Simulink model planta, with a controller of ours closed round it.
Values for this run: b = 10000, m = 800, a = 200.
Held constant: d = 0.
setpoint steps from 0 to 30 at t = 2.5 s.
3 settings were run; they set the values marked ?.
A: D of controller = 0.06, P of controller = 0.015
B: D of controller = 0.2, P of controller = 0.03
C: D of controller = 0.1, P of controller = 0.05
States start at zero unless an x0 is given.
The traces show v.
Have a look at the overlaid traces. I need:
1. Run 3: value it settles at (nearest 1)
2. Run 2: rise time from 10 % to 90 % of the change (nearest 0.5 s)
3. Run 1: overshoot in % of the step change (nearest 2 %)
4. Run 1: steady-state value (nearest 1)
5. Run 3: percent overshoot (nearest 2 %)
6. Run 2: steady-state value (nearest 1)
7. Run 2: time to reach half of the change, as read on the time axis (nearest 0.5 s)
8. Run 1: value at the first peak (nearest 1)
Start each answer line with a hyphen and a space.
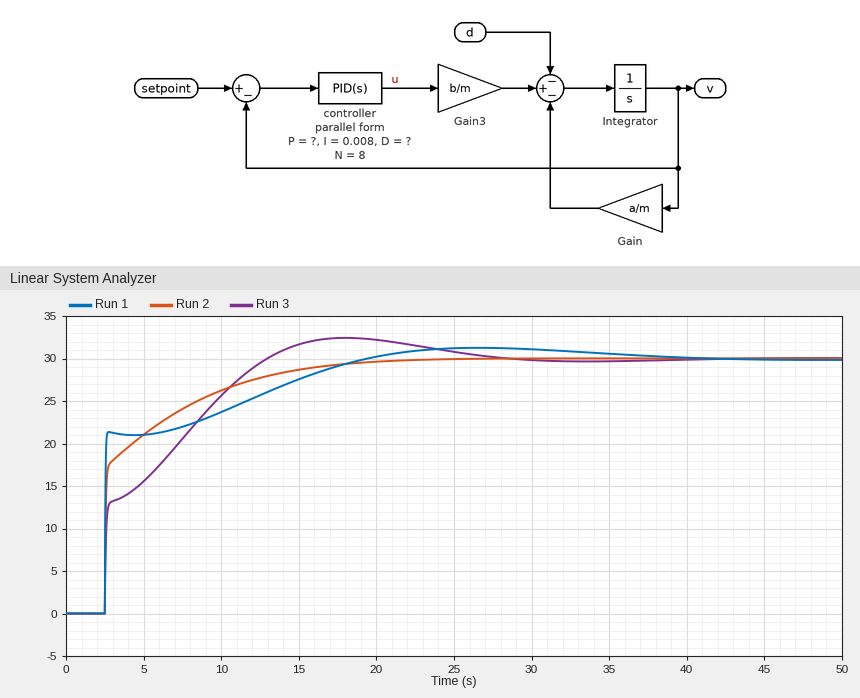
- 30
- 8.5 s
- 4 %
- 30
- 8 %
- 30
- 2.5 s
- 31
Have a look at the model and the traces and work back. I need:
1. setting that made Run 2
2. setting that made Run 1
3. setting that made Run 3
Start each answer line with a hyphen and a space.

- C
- B
- A
